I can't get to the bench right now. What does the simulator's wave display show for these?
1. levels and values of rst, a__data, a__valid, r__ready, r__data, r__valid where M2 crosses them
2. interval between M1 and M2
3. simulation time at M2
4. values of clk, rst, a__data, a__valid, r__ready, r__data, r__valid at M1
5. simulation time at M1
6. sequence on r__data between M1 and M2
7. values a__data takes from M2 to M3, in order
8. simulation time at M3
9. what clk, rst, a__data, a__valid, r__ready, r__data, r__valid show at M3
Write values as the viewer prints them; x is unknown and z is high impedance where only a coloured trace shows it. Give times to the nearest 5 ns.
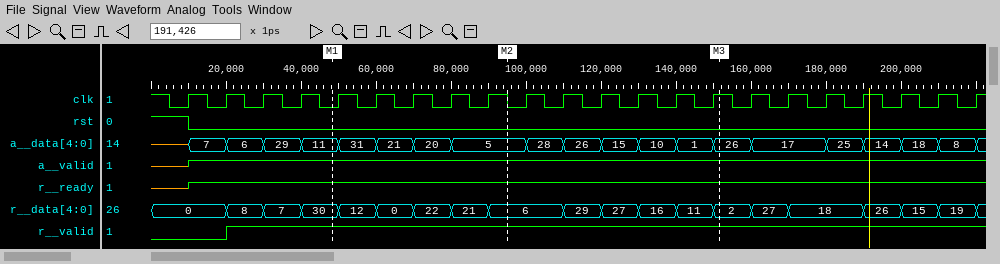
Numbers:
rst=0, a__data=5, a__valid=1, r__ready=1, r__data=6, r__valid=1
45 ns
95 ns
clk=0, rst=0, a__data=11, a__valid=1, r__ready=1, r__data=30, r__valid=1
50 ns
30, 12, 0, 22, 21, 6
5, 28, 26, 15, 10, 1, 26
150 ns
clk=1, rst=0, a__data=26, a__valid=1, r__ready=1, r__data=2, r__valid=1
